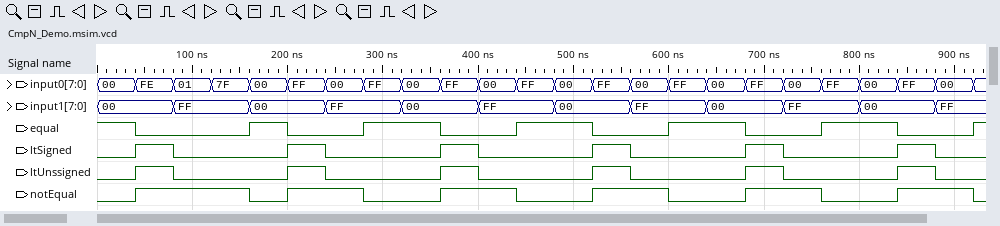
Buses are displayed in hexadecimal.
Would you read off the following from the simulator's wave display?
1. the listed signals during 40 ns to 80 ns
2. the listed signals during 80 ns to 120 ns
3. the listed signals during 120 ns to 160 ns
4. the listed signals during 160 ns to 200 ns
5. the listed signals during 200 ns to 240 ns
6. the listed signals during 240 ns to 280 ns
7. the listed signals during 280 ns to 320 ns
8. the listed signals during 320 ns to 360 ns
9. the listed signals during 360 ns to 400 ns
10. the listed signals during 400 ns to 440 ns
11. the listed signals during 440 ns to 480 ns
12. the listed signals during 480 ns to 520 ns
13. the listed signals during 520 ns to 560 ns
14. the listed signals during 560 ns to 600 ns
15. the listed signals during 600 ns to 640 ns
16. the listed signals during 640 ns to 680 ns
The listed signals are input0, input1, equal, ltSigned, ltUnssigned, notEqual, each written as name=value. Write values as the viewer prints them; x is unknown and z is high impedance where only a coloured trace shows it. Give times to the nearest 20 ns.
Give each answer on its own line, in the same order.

input0=FE, input1=00, equal=0, ltSigned=1, ltUnssigned=1, notEqual=1
input0=01, input1=FF, equal=0, ltSigned=0, ltUnssigned=0, notEqual=1
input0=7F, input1=FF, equal=0, ltSigned=0, ltUnssigned=0, notEqual=1
input0=00, input1=00, equal=1, ltSigned=0, ltUnssigned=0, notEqual=0
input0=FF, input1=00, equal=0, ltSigned=1, ltUnssigned=1, notEqual=1
input0=00, input1=FF, equal=0, ltSigned=0, ltUnssigned=0, notEqual=1
input0=FF, input1=FF, equal=1, ltSigned=0, ltUnssigned=0, notEqual=0
input0=00, input1=00, equal=1, ltSigned=0, ltUnssigned=0, notEqual=0
input0=FF, input1=00, equal=0, ltSigned=1, ltUnssigned=1, notEqual=1
input0=00, input1=FF, equal=0, ltSigned=0, ltUnssigned=0, notEqual=1
input0=FF, input1=FF, equal=1, ltSigned=0, ltUnssigned=0, notEqual=0
input0=00, input1=00, equal=1, ltSigned=0, ltUnssigned=0, notEqual=0
input0=FF, input1=00, equal=0, ltSigned=1, ltUnssigned=1, notEqual=1
input0=00, input1=FF, equal=0, ltSigned=0, ltUnssigned=0, notEqual=1
input0=FF, input1=FF, equal=1, ltSigned=0, ltUnssigned=0, notEqual=0
input0=00, input1=00, equal=1, ltSigned=0, ltUnssigned=0, notEqual=0
